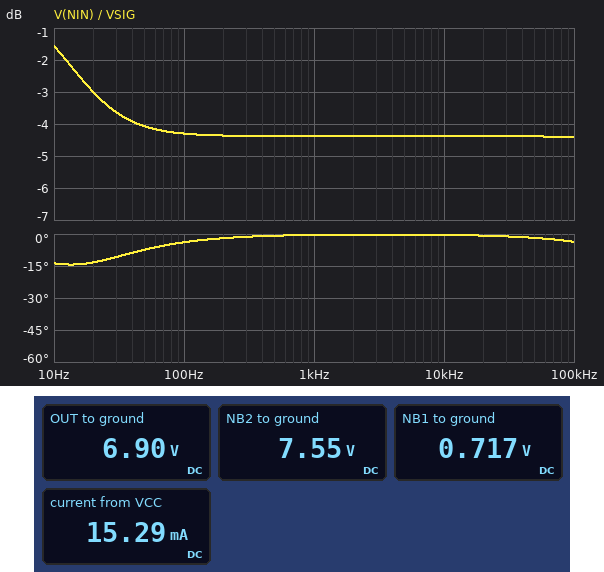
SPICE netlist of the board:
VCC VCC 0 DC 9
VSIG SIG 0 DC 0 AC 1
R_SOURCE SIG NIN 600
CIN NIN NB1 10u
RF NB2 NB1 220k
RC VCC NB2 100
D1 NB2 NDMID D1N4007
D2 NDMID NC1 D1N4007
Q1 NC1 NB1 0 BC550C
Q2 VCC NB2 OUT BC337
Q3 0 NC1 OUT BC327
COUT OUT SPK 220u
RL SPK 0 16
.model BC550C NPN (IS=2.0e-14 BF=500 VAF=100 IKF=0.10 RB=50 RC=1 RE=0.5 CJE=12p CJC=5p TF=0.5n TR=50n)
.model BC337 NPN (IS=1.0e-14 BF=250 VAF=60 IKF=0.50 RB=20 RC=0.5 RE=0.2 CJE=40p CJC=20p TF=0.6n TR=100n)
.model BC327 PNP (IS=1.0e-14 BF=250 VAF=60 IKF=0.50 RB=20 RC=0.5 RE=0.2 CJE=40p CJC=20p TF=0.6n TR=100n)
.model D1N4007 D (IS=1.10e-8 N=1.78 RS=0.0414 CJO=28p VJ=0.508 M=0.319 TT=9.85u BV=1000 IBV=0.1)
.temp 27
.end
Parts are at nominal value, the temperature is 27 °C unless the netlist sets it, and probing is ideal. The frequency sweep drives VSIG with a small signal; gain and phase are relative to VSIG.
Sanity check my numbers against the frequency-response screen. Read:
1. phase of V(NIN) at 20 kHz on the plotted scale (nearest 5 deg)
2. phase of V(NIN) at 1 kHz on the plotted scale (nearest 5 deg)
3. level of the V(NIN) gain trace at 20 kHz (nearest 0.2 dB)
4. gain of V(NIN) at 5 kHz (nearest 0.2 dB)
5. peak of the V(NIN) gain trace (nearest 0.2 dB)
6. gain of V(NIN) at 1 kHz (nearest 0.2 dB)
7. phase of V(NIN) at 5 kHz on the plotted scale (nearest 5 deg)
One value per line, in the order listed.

0 deg
0 deg
-4.4 dB
-4.4 dB
-1.6 dB
-4.4 dB
0 deg
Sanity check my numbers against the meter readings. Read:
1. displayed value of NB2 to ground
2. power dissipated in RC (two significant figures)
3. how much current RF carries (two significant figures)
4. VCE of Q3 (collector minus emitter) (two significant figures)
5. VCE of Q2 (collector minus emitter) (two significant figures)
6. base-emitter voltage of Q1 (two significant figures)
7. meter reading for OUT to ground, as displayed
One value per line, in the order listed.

7.55 V
21 mW
31 µA
-6.9 V
2.1 V
720 mV
6.90 V
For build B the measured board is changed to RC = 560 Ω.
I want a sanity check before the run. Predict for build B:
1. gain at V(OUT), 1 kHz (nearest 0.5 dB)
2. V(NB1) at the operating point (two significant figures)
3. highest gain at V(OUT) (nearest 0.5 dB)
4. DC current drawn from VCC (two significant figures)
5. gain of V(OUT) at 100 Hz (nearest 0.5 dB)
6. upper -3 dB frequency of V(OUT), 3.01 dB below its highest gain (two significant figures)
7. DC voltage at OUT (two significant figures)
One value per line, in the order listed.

26.5 dB
700 mV
32.5 dB
8.4 mA
27.0 dB
36 Hz
3.8 V
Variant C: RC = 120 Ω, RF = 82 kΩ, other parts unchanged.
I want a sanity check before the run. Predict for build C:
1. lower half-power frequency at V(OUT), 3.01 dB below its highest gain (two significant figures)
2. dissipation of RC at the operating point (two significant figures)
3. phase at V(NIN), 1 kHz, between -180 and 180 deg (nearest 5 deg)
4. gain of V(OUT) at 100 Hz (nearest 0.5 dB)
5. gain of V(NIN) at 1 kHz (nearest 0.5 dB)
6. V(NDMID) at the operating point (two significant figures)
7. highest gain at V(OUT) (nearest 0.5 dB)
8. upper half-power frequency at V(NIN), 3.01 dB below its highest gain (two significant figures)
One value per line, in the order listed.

11 Hz
81 mW
0 deg
26.0 dB
-7.5 dB
5.2 V
26.5 dB
19 Hz
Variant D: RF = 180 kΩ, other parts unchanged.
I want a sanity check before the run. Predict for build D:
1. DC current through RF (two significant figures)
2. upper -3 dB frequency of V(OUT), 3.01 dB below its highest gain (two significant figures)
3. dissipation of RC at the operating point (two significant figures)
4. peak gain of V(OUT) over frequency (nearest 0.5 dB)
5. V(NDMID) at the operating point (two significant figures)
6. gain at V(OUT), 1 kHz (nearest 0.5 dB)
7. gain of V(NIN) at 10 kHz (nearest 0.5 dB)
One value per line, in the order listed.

37 µA
370 kHz
28 mW
25.0 dB
6.7 V
22.5 dB
-5.0 dB
